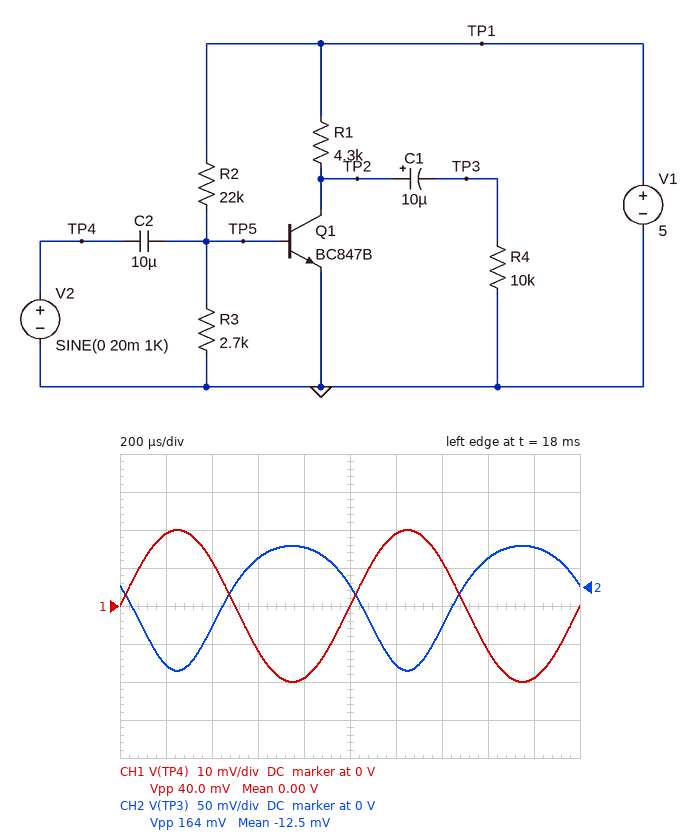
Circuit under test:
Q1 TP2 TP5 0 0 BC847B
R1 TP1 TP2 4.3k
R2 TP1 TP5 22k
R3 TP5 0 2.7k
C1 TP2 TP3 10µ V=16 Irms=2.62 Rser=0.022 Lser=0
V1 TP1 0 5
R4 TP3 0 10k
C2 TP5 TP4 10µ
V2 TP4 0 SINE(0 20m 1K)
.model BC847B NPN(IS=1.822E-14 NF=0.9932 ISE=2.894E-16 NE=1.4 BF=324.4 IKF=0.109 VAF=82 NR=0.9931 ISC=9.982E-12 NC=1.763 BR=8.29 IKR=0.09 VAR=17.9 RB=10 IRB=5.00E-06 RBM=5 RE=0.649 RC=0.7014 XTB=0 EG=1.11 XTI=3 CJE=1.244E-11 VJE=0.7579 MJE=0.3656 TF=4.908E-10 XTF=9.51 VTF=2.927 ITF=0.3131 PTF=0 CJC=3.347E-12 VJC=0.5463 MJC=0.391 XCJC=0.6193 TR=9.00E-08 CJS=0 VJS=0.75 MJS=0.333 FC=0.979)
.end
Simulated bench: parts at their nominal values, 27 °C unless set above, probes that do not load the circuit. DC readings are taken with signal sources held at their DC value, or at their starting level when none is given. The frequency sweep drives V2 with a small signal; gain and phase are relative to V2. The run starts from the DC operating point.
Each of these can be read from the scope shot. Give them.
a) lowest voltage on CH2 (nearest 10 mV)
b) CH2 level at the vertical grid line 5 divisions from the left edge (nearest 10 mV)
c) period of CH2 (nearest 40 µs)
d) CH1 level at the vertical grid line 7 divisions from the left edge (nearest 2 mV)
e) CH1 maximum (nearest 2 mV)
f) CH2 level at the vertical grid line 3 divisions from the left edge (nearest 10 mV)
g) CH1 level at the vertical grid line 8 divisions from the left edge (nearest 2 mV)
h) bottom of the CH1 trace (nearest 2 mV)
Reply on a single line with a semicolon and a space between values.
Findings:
-110 mV; 0 V; 1.00 ms; 12 mV; 20 mV; 40 mV; -12 mV; -20 mV
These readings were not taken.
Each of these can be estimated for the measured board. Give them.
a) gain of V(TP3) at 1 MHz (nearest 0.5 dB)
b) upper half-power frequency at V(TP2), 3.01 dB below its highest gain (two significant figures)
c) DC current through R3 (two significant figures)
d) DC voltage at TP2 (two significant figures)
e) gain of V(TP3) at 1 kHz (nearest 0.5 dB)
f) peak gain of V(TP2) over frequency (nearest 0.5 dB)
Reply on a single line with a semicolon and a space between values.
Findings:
11.5 dB; 40 MHz; 200 µA; 4.9 V; 11.5 dB; 11.5 dB
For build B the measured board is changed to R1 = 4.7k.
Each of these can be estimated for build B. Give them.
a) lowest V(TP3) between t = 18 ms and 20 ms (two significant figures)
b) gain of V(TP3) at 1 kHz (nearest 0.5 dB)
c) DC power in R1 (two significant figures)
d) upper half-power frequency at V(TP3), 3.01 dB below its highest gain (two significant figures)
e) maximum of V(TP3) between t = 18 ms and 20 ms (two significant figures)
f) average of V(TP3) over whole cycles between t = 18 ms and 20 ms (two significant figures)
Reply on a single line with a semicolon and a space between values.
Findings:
-120 mV; 12.0 dB; 4.8 µW; 37 MHz; 57 mV; -14 mV
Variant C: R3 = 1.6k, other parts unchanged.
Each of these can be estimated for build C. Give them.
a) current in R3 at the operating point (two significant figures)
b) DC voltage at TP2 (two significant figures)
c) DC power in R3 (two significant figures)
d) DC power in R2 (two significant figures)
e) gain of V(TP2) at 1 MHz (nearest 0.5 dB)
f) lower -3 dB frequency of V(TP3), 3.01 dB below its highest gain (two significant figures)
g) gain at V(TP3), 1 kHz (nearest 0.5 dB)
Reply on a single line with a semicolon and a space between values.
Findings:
210 µA; 5.0 V; 72 µW; 990 µW; -31.5 dB; 36 MHz; -58.5 dB
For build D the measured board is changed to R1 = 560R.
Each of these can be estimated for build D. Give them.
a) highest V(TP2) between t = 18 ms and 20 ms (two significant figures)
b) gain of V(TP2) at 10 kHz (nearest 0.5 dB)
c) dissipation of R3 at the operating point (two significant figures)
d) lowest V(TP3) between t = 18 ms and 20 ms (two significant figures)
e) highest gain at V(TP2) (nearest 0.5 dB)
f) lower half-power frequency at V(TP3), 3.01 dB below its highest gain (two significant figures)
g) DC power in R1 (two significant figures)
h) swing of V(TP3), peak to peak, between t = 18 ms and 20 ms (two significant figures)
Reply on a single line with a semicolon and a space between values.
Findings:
5.0 V; -3.5 dB; 110 µW; -19 mV; -1.0 dB; 22 Hz; 580 nW; 29 mV
